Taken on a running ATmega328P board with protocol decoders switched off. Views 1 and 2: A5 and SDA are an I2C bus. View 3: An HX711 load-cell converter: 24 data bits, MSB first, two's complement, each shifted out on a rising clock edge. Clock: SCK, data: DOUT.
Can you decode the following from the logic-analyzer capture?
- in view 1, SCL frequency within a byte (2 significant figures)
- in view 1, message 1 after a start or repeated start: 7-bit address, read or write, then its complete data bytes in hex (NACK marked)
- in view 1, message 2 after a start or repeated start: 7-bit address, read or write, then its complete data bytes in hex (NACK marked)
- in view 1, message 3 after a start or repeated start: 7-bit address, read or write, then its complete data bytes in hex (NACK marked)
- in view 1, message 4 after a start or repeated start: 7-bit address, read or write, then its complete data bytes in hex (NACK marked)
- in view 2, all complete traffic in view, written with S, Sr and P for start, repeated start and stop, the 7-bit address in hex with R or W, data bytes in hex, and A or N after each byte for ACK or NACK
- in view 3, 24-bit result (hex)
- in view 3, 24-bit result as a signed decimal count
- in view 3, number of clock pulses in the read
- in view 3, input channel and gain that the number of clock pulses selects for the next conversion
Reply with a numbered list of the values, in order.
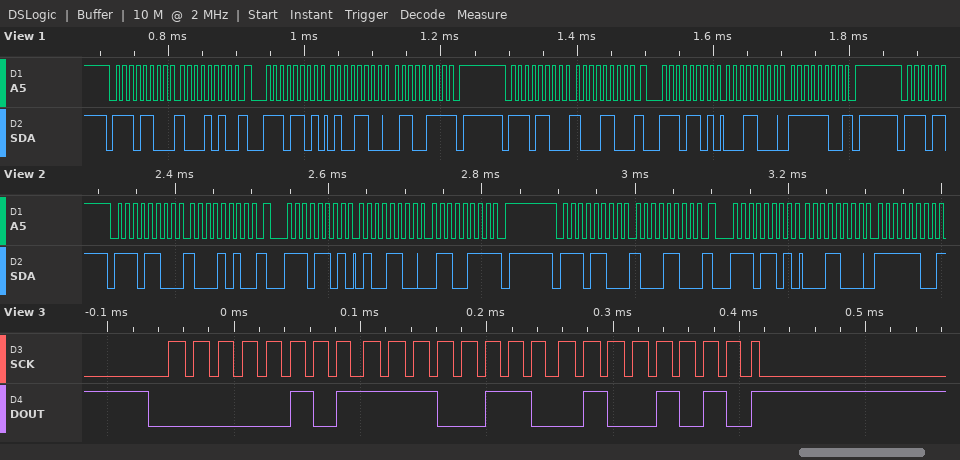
1. 100 kHz
2. 0x76 write: 8A
3. 0x76 read: 4C 67 NACK
4. 0x76 write: 8C
5. 0x76 read: 18 FC NACK
6. S 76W A 8A A Sr 76R A 4C A 67 N P S 76W A 8C A Sr 76R A 18 A FC N
7. 0x05E64A
8. 386634
9. 25
10. channel A, gain 128
